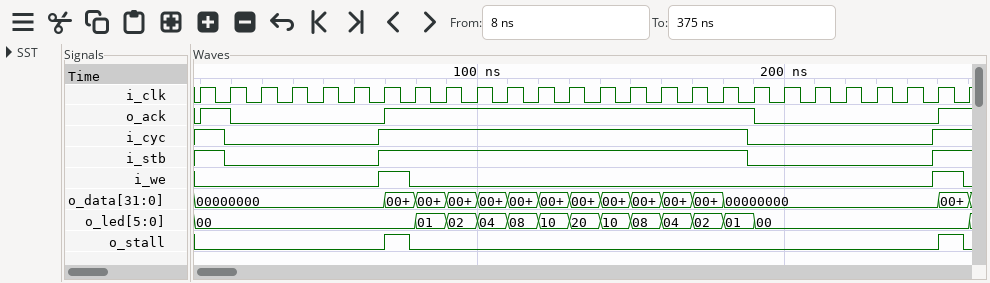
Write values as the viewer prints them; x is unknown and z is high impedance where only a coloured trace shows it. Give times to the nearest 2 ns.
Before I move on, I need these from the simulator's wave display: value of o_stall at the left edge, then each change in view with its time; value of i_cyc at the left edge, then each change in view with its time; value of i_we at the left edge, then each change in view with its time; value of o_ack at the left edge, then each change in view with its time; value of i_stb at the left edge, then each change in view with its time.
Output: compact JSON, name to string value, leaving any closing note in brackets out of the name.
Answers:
{"value of o_stall at the left edge, then each change in view with its time": "0, 1 at 70 ns, 0 at 78 ns, 1 at 250 ns, 0 at 258 ns", "value of i_cyc at the left edge, then each change in view with its time": "1, 0 at 18 ns, 1 at 68 ns, 0 at 188 ns, 1 at 248 ns", "value of i_we at the left edge, then each change in view with its time": "0, 1 at 68 ns, 0 at 78 ns, 1 at 248 ns, 0 at 258 ns", "value of o_ack at the left edge, then each change in view with its time": "0, 1 at 10 ns, 0 at 20 ns, 1 at 70 ns, 0 at 190 ns, 1 at 250 ns", "value of i_stb at the left edge, then each change in view with its time": "1, 0 at 18 ns, 1 at 68 ns, 0 at 188 ns, 1 at 248 ns"}
